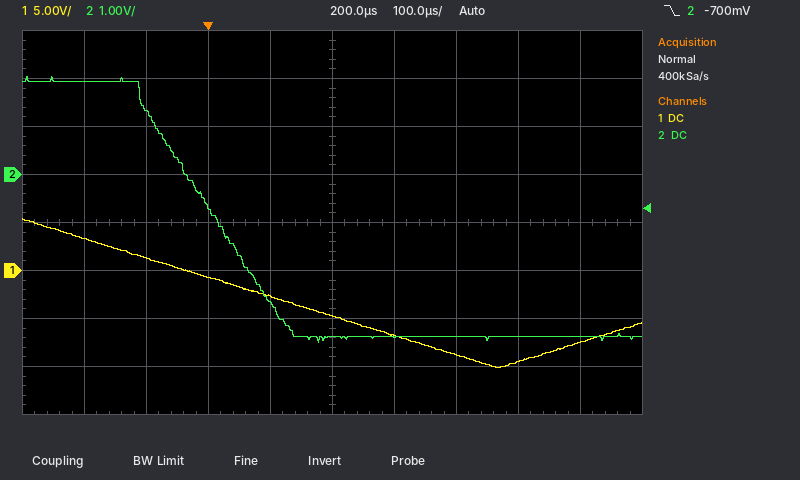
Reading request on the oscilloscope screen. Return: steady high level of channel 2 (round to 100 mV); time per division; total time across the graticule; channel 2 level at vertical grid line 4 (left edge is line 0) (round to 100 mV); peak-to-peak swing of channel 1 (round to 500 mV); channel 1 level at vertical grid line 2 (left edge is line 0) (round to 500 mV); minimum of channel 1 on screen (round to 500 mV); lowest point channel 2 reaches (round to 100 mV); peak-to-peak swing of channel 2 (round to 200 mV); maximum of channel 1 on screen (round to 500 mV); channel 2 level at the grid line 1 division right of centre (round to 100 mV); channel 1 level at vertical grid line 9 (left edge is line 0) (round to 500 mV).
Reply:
1.9 V
100 µs
1 ms
-2.7 V
15.5 V
1.5 V
-10.0 V
-3.5 V
5.6 V
5.5 V
-3.4 V
-7.5 V
